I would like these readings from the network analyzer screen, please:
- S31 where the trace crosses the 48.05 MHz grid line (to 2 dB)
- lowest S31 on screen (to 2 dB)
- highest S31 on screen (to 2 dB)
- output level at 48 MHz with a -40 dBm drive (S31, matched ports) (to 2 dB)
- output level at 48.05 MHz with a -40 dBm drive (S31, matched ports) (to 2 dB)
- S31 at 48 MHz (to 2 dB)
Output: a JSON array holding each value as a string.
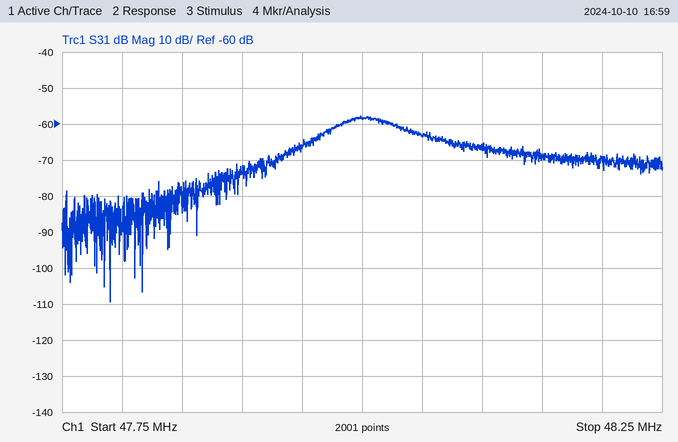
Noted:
["-64 dB", "-110 dB", "-58 dB", "-98 dBm", "-104 dBm", "-58 dB"]
